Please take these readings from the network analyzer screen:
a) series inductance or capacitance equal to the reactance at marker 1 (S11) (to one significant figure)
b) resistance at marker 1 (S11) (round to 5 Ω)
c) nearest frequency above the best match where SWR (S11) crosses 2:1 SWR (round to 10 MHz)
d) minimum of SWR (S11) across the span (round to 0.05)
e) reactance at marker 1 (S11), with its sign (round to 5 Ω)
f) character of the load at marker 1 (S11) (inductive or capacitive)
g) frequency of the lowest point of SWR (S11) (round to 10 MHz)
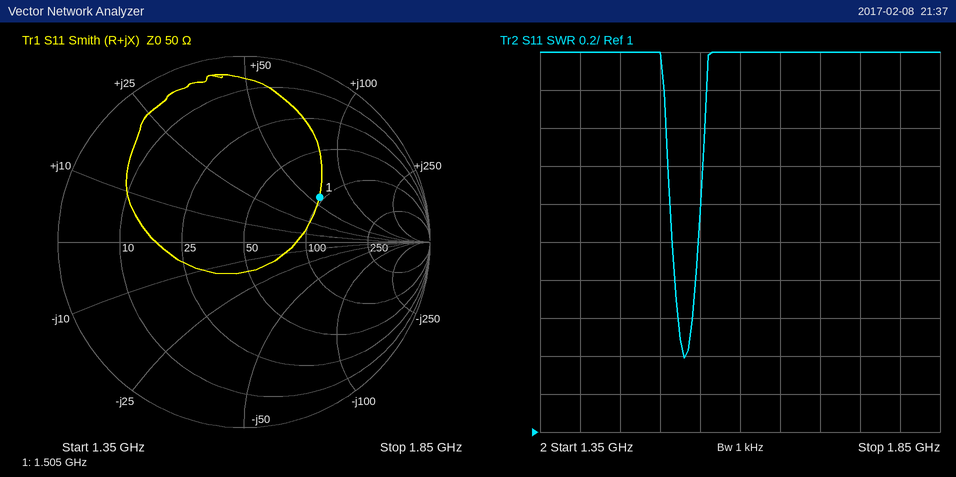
6 nH
95 Ω
1.55 GHz
1.40
+60 Ω
inductive
1.53 GHz
